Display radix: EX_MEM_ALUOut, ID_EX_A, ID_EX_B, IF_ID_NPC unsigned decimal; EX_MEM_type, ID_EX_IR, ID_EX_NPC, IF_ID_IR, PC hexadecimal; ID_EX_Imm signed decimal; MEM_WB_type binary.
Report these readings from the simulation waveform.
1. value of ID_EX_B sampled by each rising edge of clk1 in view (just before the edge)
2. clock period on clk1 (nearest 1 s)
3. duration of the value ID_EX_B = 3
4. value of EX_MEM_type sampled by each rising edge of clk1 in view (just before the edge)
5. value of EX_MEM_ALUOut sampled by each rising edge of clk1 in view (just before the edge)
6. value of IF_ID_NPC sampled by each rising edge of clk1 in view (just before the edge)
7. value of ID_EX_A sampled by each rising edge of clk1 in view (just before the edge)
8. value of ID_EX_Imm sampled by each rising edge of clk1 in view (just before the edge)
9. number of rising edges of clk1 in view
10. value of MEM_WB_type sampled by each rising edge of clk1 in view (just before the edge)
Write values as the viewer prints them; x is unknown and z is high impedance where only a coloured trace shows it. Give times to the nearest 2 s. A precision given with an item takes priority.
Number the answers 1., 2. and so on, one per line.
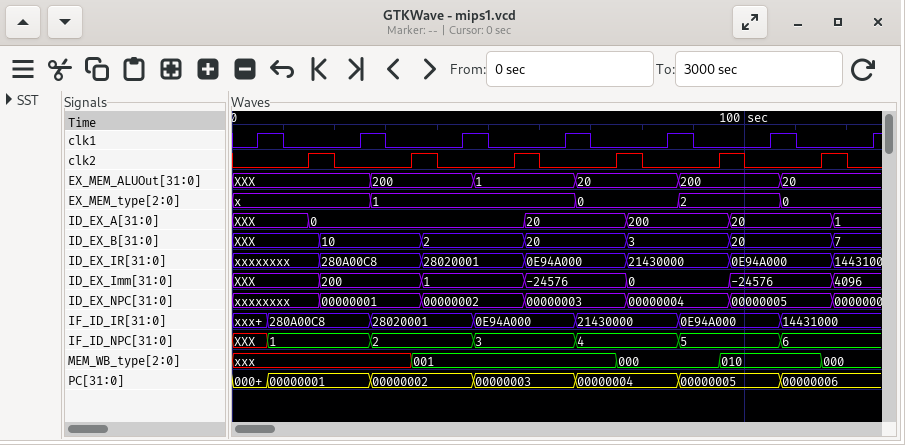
1. XXX, 10, 2, 20, 3, 20, 7
2. 20 s
3. 20 s
4. x, x, 1, 1, 0, 2, 0
5. XXX, XXX, 200, 1, 20, 200, 20
6. XXX, 1, 2, 3, 4, 5, 6
7. XXX, 0, 0, 20, 200, 20, 1
8. XXX, 200, 1, -24576, 0, -24576, 4096
9. 7
10. xxx, xxx, 001, 001, 000, 010, 000
